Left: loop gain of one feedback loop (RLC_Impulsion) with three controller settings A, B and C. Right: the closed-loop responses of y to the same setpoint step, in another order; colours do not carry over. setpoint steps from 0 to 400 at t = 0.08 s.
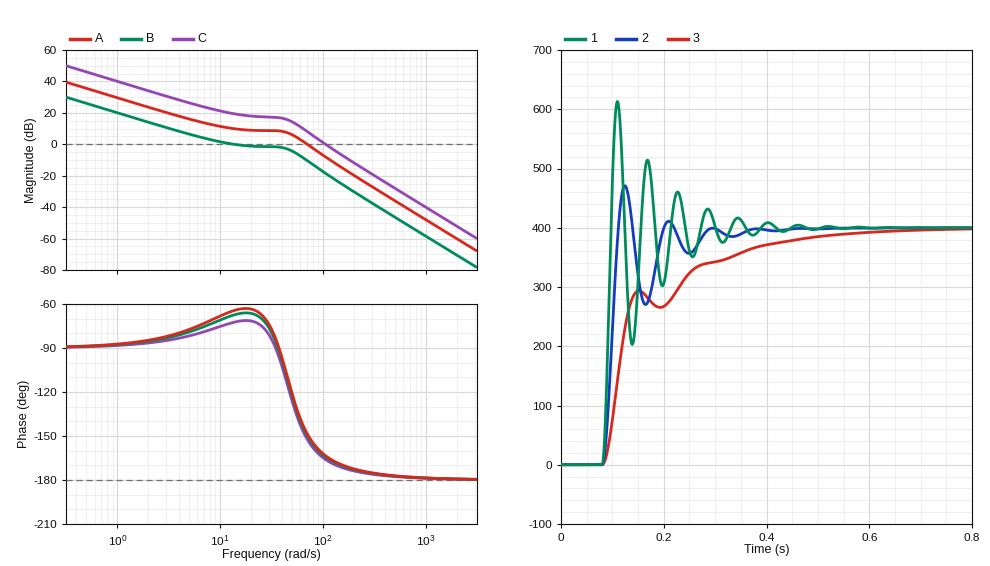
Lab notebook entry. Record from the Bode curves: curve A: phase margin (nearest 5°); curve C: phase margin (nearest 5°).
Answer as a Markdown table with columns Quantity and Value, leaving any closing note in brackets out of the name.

| Quantity | Value |
|---|---|
| curve A: phase margin | 30° |
| curve C: phase margin | 15° |
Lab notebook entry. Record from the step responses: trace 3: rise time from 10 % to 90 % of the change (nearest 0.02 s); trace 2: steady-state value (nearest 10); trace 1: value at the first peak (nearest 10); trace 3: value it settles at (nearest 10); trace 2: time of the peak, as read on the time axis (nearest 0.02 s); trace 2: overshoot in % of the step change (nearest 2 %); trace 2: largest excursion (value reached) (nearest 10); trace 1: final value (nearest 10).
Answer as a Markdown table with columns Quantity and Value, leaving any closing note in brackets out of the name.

| Quantity | Value |
|---|---|
| trace 3: rise time from 10 % to 90 % of the change | 0.26 s |
| trace 2: steady-state value | 400 |
| trace 1: value at the first peak | 610 |
| trace 3: value it settles at | 400 |
| trace 2: time of the peak, as read on the time axis | 0.12 s |
| trace 2: overshoot in % of the step change | 18 % |
| trace 2: largest excursion (value reached) | 470 |
| trace 1: final value | 400 |
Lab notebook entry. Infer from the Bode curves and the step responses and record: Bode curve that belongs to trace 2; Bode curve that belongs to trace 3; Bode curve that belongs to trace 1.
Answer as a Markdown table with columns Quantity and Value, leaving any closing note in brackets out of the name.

| Quantity | Value |
|---|---|
| Bode curve that belongs to trace 2 | A |
| Bode curve that belongs to trace 3 | B |
| Bode curve that belongs to trace 1 | C |
